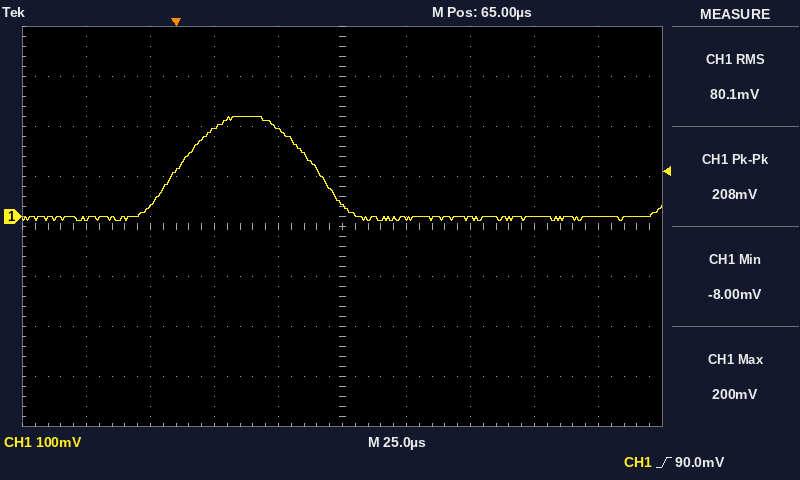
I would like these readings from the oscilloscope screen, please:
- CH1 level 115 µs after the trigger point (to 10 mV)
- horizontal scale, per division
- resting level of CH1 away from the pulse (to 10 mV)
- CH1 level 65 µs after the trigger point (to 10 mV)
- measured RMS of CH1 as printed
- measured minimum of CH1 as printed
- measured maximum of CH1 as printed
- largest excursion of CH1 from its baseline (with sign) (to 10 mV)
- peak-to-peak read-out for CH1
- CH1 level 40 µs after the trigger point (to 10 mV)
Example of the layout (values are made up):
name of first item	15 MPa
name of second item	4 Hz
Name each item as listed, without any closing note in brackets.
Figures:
CH1 level 115 µs after the trigger point	0 mV
horizontal scale, per division	25 µs
resting level of CH1 away from the pulse	0 mV
CH1 level 65 µs after the trigger point	20 mV
measured RMS of CH1 as printed	80.1 mV
measured minimum of CH1 as printed	-8.00 mV
measured maximum of CH1 as printed	200 mV
largest excursion of CH1 from its baseline (with sign)	+200 mV
peak-to-peak read-out for CH1	208 mV
CH1 level 40 µs after the trigger point	170 mV
